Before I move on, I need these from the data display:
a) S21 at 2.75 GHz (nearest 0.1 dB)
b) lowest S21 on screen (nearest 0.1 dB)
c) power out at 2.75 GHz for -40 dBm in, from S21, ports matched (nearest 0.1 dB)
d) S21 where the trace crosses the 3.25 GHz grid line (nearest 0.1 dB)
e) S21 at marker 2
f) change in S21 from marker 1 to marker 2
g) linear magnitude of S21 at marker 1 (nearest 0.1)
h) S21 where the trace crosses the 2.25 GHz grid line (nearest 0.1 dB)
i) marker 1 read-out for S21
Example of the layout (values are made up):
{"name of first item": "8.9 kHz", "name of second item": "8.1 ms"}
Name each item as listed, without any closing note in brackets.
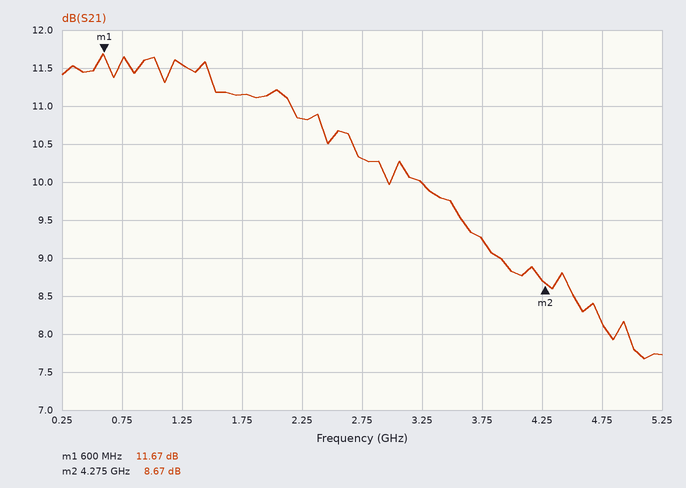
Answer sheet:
{"S21 at 2.75 GHz": "10.3 dB", "lowest S21 on screen": "7.7 dB", "power out at 2.75 GHz for -40 dBm in, from S21, ports matched": "-29.7 dBm", "S21 where the trace crosses the 3.25 GHz grid line": "10.0 dB", "S21 at marker 2": "8.67 dB", "change in S21 from marker 1 to marker 2": "-3.00 dB", "linear magnitude of S21 at marker 1": "3.8", "S21 where the trace crosses the 2.25 GHz grid line": "10.8 dB", "marker 1 read-out for S21": "11.67 dB"}
